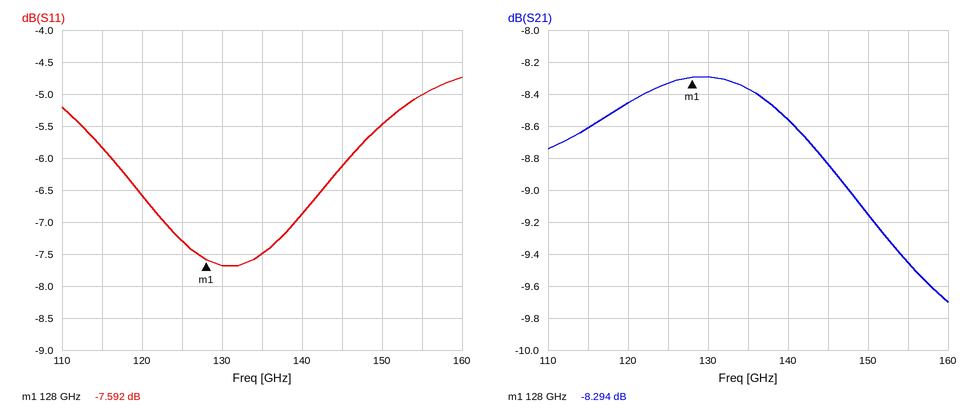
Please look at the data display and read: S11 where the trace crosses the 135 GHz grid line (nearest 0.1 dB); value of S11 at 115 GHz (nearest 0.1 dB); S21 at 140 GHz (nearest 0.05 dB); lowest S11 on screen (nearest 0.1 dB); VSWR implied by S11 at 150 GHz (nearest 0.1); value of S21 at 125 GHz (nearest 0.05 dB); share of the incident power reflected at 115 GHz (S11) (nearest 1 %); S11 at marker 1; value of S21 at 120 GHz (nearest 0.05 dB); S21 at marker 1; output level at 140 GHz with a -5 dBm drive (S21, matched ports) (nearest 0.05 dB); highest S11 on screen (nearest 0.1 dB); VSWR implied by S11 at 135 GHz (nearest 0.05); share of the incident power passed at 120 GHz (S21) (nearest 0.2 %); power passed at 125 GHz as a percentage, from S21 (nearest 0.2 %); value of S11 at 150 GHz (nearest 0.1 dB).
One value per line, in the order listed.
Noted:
-7.5 dB
-5.8 dB
-8.55 dB
-7.7 dB
3.3
-8.35 dB
26 %
-7.592 dB
-8.45 dB
-8.294 dB
-13.55 dBm
-4.7 dB
2.45
14.2 %
14.6 %
-5.5 dB
